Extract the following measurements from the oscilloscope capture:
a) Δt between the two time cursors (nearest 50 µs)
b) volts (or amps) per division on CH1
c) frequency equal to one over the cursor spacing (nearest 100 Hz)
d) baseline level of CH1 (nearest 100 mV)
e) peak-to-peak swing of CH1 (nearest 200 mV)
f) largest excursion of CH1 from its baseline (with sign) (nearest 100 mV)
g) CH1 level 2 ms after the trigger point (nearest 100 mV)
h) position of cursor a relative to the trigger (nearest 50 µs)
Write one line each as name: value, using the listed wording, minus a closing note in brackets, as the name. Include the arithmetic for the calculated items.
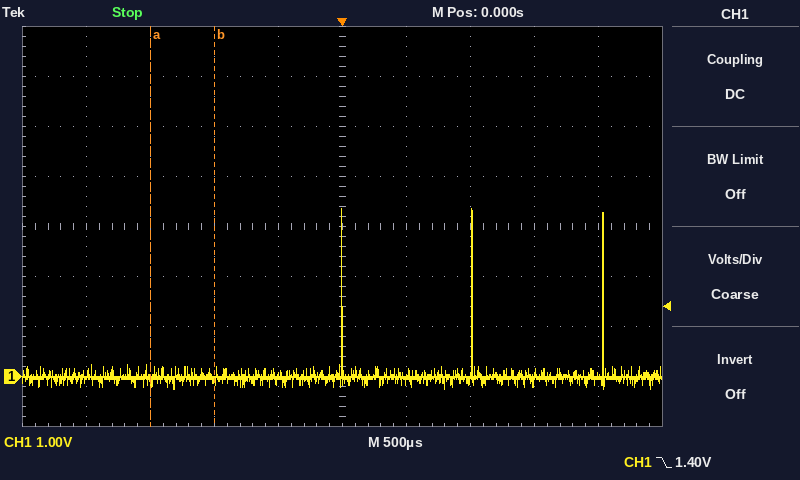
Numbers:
Δt between the two time cursors: 500 µs
volts (or amps) per division on CH1: 1 V
frequency equal to one over the cursor spacing: 1 / 500 µs ≈ 2.0 kHz
baseline level of CH1: 0.0 V
peak-to-peak swing of CH1: 3.6 V
largest excursion of CH1 from its baseline (with sign): +3.4 V
CH1 level 2 ms after the trigger point: 0.0 V
position of cursor a relative to the trigger: -1.50 ms
